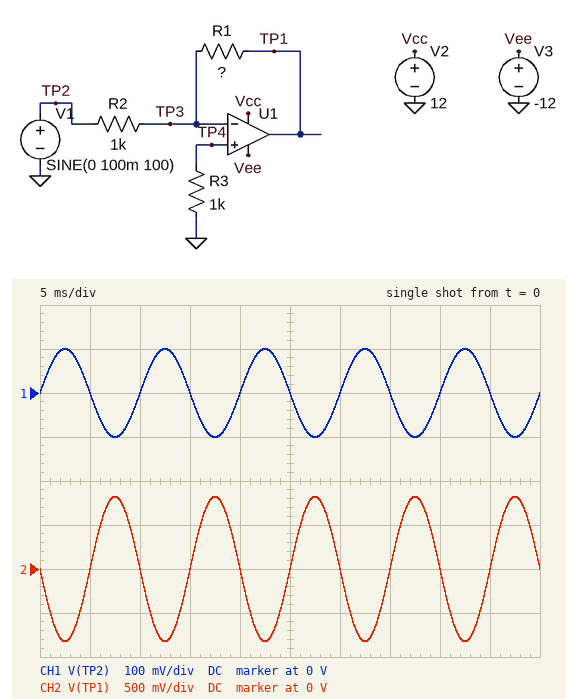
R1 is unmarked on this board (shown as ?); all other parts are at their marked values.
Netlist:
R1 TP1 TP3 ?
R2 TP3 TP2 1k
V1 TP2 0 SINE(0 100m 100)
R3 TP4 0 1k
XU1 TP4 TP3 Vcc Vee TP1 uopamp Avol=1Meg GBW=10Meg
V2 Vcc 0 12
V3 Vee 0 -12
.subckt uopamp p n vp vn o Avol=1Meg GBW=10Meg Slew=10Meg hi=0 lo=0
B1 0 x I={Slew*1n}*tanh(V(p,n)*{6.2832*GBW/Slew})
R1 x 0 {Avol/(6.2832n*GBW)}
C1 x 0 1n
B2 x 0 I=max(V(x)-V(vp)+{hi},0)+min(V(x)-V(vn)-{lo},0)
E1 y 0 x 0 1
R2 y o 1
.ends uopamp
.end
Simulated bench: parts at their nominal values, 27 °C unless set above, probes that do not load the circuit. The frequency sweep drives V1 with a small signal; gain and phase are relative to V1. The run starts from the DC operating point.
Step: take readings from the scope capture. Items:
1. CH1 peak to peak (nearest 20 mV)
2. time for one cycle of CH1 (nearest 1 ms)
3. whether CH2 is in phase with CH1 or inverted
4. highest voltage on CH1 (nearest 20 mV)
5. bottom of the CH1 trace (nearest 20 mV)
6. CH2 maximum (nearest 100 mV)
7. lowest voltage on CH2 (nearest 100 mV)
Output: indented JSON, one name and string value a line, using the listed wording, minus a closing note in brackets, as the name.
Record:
{
  "CH1 peak to peak": "200 mV",
  "time for one cycle of CH1": "10 ms",
  "whether CH2 is in phase with CH1 or inverted": "inverted",
  "highest voltage on CH1": "100 mV",
  "bottom of the CH1 trace": "-100 mV",
  "CH2 maximum": "800 mV",
  "lowest voltage on CH2": "-800 mV"
}
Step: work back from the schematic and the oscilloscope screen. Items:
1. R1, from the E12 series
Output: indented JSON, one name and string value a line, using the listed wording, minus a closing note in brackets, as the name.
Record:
{
  "R1, from the E12 series": "8.2 kΩ"
}
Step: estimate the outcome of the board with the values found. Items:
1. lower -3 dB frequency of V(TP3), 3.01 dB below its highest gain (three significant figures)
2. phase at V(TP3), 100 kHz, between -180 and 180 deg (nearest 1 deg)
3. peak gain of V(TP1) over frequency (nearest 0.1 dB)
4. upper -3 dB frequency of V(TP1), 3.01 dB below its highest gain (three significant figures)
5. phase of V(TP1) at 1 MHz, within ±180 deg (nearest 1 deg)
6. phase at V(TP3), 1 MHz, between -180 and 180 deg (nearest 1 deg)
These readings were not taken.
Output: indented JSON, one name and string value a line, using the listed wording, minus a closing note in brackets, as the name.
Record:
{
  "lower -3 dB frequency of V(TP3), 3.01 dB below its highest gain": "1.09 MHz",
  "phase at V(TP3), 100 kHz, between -180 and 180 deg": "85 deg",
  "peak gain of V(TP1) over frequency": "18.3 dB",
  "upper -3 dB frequency of V(TP1), 3.01 dB below its highest gain": "1.09 MHz",
  "phase of V(TP1) at 1 MHz, within ±180 deg": "137 deg",
  "phase at V(TP3), 1 MHz, between -180 and 180 deg": "47 deg"
}
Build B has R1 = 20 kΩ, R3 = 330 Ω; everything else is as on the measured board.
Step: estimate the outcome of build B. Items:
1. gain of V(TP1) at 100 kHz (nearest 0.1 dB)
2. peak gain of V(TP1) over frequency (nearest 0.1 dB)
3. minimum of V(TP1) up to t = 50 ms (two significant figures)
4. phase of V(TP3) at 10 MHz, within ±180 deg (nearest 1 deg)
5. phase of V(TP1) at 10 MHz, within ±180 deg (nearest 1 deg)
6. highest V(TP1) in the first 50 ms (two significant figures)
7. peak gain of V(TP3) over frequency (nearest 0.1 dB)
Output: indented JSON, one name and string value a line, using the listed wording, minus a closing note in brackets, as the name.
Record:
{
  "gain of V(TP1) at 100 kHz": "25.8 dB",
  "peak gain of V(TP1) over frequency": "26.0 dB",
  "minimum of V(TP1) up to t = 50 ms": "-2.0 V",
  "phase of V(TP3) at 10 MHz, within ±180 deg": "3 deg",
  "phase of V(TP1) at 10 MHz, within ±180 deg": "93 deg",
  "highest V(TP1) in the first 50 ms": "2.0 V",
  "peak gain of V(TP3) over frequency": "-0.4 dB"
}
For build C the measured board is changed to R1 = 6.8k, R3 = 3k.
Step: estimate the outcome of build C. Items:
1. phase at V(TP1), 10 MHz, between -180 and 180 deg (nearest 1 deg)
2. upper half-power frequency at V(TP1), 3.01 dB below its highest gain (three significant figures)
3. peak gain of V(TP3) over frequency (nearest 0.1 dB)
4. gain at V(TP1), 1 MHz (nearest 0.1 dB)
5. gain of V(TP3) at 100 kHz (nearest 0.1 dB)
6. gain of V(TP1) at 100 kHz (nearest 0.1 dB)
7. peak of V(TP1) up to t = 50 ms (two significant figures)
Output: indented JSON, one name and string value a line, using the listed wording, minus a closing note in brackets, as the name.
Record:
{
  "phase at V(TP1), 10 MHz, between -180 and 180 deg": "97 deg",
  "upper half-power frequency at V(TP1), 3.01 dB below its highest gain": "1.28 MHz",
  "peak gain of V(TP3) over frequency": "-1.2 dB",
  "gain at V(TP1), 1 MHz": "14.6 dB",
  "gain of V(TP3) at 100 kHz": "-23.4 dB",
  "gain of V(TP1) at 100 kHz": "16.6 dB",
  "peak of V(TP1) up to t = 50 ms": "680 mV"
}
